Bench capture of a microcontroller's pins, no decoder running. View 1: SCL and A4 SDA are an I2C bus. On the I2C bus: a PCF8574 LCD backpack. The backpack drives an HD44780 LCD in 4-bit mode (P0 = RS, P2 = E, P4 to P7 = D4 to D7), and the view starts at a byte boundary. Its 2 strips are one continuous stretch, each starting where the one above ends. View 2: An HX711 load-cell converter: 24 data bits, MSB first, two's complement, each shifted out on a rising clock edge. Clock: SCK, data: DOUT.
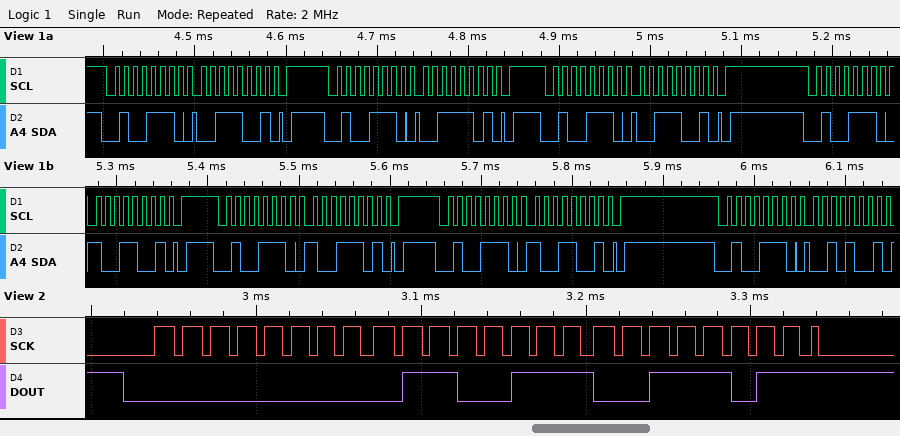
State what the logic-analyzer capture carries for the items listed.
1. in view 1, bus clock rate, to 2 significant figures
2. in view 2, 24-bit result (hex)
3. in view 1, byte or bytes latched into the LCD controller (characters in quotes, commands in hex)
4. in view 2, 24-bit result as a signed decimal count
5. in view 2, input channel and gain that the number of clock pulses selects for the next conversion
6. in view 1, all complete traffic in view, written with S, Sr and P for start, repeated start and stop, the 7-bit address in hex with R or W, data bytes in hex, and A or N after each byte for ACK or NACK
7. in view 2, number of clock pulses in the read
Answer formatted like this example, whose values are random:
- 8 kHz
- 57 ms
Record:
- 100 kHz
- 0x00673B
- '9'
- 26427
- channel A, gain 128
- S 27W A 39 A P S 27W A 3D A P S 27W A 39 A P S 27W A 99 A P S 27W A 9D A P S 27W A 99 A P S 27W A 29 A
- 25
